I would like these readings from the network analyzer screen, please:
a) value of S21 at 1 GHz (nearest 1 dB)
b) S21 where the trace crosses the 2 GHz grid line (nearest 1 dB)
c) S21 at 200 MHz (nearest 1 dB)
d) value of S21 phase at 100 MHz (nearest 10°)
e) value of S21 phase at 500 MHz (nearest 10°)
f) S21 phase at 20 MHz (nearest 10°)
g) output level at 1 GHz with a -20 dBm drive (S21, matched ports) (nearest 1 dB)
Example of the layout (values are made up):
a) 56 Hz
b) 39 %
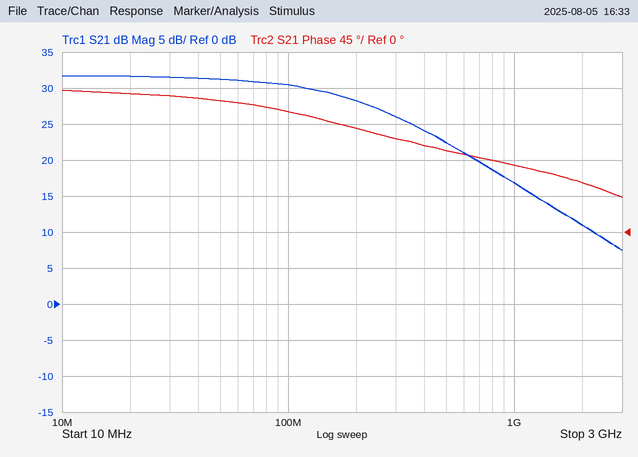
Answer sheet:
a) 17 dB
b) 11 dB
c) 28 dB
d) 150°
e) 100°
f) 170°
g) -3 dBm
